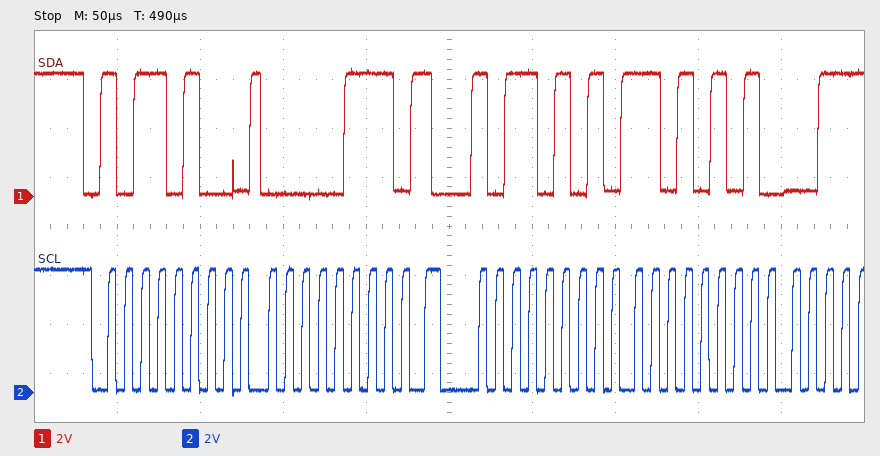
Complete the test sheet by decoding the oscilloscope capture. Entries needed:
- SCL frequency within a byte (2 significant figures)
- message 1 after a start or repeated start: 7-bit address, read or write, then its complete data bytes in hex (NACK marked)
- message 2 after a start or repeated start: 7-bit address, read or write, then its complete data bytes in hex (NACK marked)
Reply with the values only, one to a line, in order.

100 kHz
0x5A write: 07
0x5A read: D5
